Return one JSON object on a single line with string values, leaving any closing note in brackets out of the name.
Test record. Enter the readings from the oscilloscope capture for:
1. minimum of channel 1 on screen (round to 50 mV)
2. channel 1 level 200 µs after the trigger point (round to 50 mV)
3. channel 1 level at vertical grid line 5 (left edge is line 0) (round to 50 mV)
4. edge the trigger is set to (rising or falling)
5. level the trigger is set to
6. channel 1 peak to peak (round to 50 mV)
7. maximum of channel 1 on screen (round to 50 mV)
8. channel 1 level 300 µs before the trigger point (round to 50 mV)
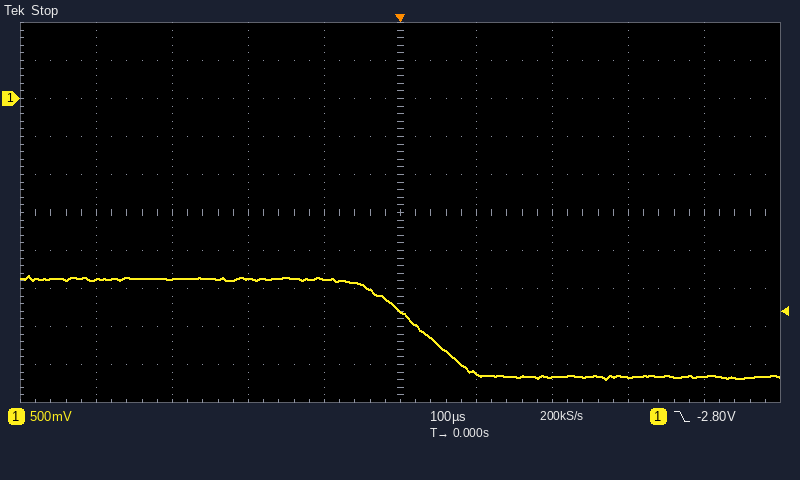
{"minimum of channel 1 on screen": "-3.70 V", "channel 1 level 200 µs after the trigger point": "-3.65 V", "channel 1 level at vertical grid line 5 (left edge is line 0)": "-2.80 V", "edge the trigger is set to": "falling", "level the trigger is set to": "-2.80 V", "channel 1 peak to peak": "1.35 V", "maximum of channel 1 on screen": "-2.35 V", "channel 1 level 300 µs before the trigger point": "-2.40 V"}
